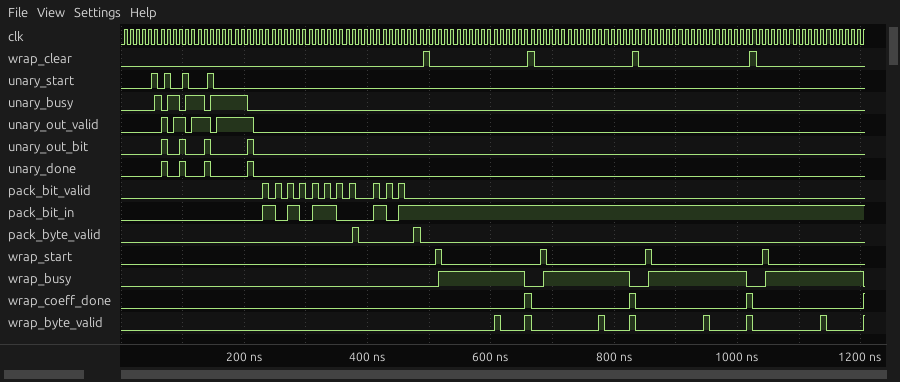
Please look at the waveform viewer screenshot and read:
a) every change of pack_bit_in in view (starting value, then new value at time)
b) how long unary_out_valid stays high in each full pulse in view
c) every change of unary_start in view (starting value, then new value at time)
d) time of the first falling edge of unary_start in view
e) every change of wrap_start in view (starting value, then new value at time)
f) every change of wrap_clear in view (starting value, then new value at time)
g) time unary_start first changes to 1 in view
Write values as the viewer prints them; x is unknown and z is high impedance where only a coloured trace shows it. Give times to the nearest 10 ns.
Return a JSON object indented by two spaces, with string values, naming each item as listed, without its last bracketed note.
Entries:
{
  "every change of pack_bit_in in view": "0, 1 at 230 ns, 0 at 250 ns, 1 at 270 ns, 0 at 290 ns, 1 at 310 ns, 0 at 350 ns, 1 at 410 ns, 0 at 430 ns, 1 at 450 ns",
  "how long unary_out_valid stays high in each full pulse in view": "10 ns, 20 ns, 30 ns, 60 ns",
  "every change of unary_start in view": "0, 1 at 50 ns, 0 at 60 ns, 1 at 70 ns, 0 at 80 ns, 1 at 100 ns, 0 at 110 ns, 1 at 140 ns, 0 at 150 ns",
  "time of the first falling edge of unary_start in view": "60 ns",
  "every change of wrap_start in view": "0, 1 at 510 ns, 0 at 520 ns, 1 at 680 ns, 0 at 690 ns, 1 at 850 ns, 0 at 860 ns, 1 at 1040 ns, 0 at 1050 ns",
  "every change of wrap_clear in view": "0, 1 at 490 ns, 0 at 500 ns, 1 at 660 ns, 0 at 670 ns, 1 at 830 ns, 0 at 840 ns, 1 at 1020 ns, 0 at 1030 ns",
  "time unary_start first changes to 1 in view": "50 ns"
}
